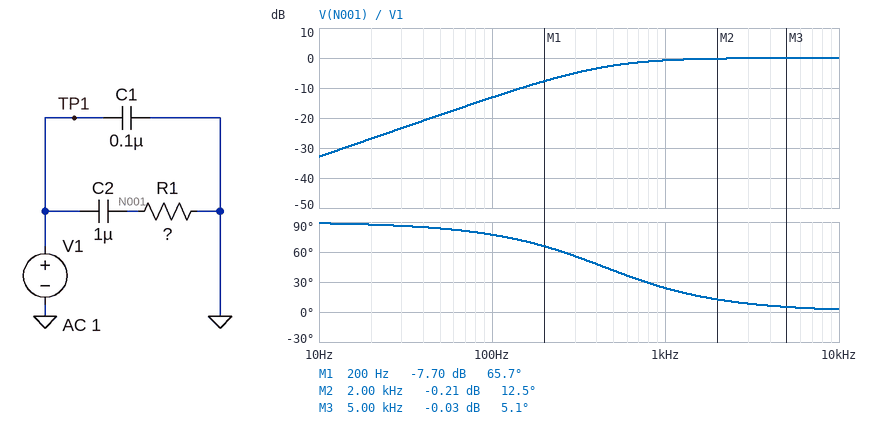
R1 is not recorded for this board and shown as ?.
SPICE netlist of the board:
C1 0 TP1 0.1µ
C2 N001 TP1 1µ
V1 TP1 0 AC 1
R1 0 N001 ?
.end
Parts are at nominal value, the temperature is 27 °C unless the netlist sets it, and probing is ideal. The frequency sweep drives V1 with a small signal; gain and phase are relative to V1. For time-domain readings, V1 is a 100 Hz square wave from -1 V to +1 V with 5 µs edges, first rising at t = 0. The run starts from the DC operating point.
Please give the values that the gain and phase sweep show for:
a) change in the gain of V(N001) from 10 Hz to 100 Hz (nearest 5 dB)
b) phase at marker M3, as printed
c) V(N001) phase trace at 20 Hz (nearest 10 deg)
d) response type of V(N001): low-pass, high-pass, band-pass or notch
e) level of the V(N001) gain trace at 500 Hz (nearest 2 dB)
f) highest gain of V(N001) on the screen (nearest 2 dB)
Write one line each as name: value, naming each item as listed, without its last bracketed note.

change in the gain of V(N001) from 10 Hz to 100 Hz: 20 dB
phase at marker M3, as printed: 5.1 deg
V(N001) phase trace at 20 Hz: 90 deg
response type of V(N001): low-pass, high-pass, band-pass or notch: high-pass
level of the V(N001) gain trace at 500 Hz: -2 dB
highest gain of V(N001) on the screen: 0 dB
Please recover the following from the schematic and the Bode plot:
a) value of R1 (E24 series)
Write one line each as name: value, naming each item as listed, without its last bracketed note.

value of R1: 360 Ω
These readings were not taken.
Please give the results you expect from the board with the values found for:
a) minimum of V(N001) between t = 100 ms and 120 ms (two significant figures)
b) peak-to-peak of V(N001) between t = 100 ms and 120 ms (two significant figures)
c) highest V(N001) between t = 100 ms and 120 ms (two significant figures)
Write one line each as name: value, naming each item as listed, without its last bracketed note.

minimum of V(N001) between t = 100 ms and 120 ms: -2.0 V
peak-to-peak of V(N001) between t = 100 ms and 120 ms: 4.0 V
highest V(N001) between t = 100 ms and 120 ms: 2.0 V
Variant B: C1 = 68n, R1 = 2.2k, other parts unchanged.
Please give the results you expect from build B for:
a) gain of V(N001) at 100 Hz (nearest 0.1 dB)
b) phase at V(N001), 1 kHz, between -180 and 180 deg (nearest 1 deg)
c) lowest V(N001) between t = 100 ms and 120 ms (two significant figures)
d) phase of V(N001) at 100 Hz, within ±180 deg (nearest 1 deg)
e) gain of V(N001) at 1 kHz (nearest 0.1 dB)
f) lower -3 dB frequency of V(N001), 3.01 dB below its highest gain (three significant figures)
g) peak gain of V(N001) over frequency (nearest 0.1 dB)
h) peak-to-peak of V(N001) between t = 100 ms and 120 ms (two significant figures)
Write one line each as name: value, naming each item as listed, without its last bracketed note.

gain of V(N001) at 100 Hz: -1.8 dB
phase at V(N001), 1 kHz, between -180 and 180 deg: 4 deg
lowest V(N001) between t = 100 ms and 120 ms: -1.8 V
phase of V(N001) at 100 Hz, within ±180 deg: 36 deg
gain of V(N001) at 1 kHz: 0 dB
lower -3 dB frequency of V(N001), 3.01 dB below its highest gain: 72.3 Hz
peak gain of V(N001) over frequency: 0 dB
peak-to-peak of V(N001) between t = 100 ms and 120 ms: 3.6 V
